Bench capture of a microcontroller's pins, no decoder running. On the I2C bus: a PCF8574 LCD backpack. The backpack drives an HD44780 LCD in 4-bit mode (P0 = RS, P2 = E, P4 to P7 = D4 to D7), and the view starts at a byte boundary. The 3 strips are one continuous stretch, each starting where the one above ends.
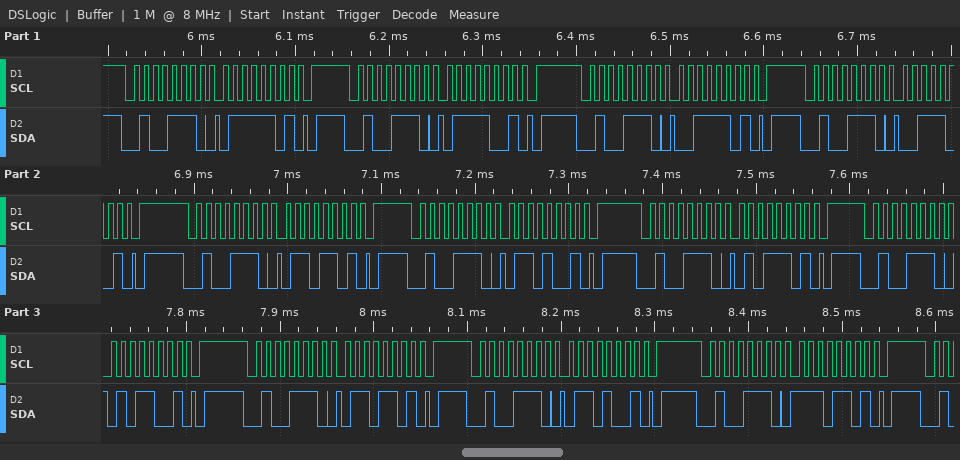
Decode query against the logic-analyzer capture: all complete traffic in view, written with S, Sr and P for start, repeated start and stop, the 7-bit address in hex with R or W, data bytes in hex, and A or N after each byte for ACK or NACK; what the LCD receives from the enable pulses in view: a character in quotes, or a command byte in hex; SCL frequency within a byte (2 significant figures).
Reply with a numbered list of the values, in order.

1. S 27W A 7D A P S 27W A 79 A P S 27W A 3D A P S 27W A 39 A P S 27W A 6D A P S 27W A 69 A P S 27W A 5D A P S 27W A 59 A P S 27W A 6D A P S 27W A 69 A P S 27W A ED A P
2. 's' 'e'
3. 100 kHz
